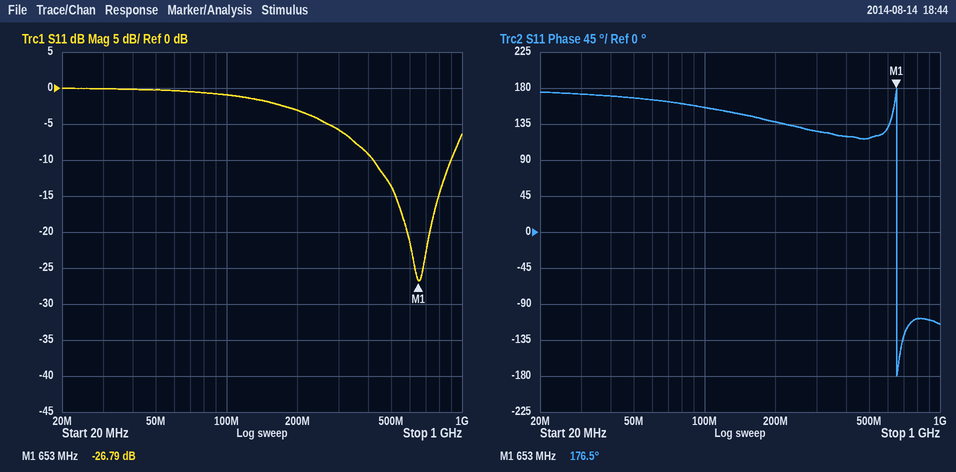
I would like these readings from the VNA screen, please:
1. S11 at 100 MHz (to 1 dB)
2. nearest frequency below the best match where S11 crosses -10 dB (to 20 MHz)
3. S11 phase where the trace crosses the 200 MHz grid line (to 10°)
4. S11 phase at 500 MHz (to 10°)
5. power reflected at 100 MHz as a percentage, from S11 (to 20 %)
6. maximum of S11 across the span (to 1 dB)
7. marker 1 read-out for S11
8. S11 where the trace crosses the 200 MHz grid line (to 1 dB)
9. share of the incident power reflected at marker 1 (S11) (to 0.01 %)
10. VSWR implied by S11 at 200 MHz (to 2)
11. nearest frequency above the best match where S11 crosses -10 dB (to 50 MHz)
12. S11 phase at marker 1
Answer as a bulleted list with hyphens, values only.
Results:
- -1 dB
- 420 MHz
- 140°
- 120°
- 80 %
- 0 dB
- -26.79 dB
- -3 dB
- 0.21 %
- 6
- 900 MHz
- 176.5°
